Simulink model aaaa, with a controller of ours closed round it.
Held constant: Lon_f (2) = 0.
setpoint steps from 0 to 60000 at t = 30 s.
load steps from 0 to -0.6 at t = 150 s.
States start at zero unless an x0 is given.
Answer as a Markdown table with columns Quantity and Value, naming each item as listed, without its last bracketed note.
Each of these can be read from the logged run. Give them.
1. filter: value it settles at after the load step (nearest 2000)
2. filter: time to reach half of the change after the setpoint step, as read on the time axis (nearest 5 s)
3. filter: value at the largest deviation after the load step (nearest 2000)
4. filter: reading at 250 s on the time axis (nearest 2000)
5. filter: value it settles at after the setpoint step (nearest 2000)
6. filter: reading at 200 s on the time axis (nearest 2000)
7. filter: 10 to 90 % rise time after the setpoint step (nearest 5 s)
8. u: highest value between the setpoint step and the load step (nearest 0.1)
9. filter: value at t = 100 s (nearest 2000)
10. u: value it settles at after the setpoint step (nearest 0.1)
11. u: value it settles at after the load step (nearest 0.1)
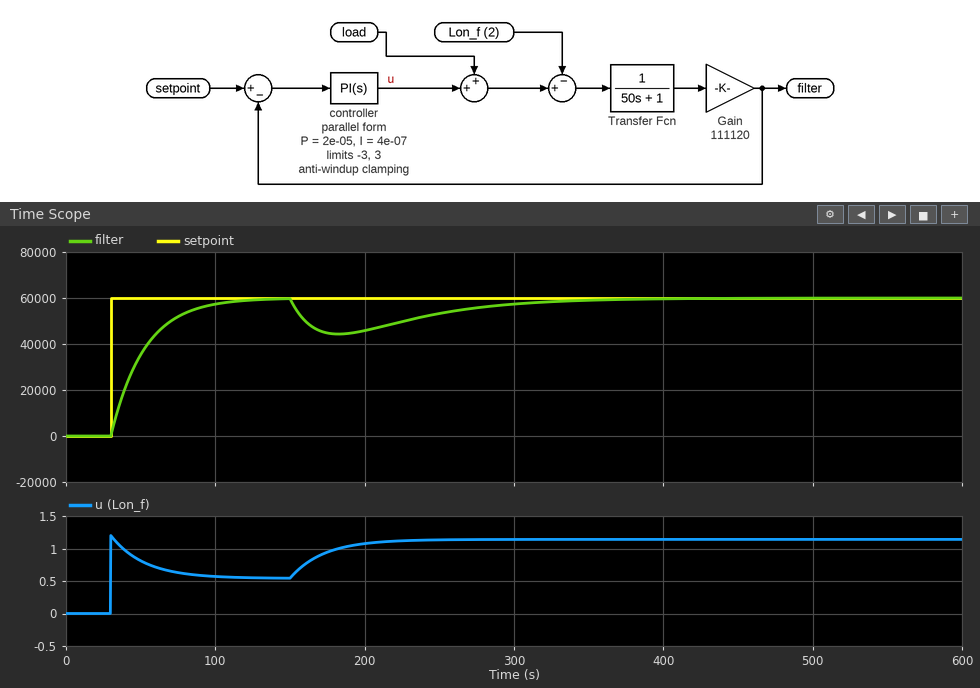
| Quantity | Value |
|---|---|
| filter: value it settles at after the load step | 60000 |
| filter: time to reach half of the change after the setpoint step, as read on the time axis | 45 s |
| filter: value at the largest deviation after the load step | 44000 |
| filter: reading at 250 s on the time axis | 54000 |
| filter: value it settles at after the setpoint step | 60000 |
| filter: reading at 200 s on the time axis | 46000 |
| filter: 10 to 90 % rise time after the setpoint step | 50 s |
| u: highest value between the setpoint step and the load step | 1.2 |
| filter: value at t = 100 s | 58000 |
| u: value it settles at after the setpoint step | 0.5 |
| u: value it settles at after the load step | 1.1 |
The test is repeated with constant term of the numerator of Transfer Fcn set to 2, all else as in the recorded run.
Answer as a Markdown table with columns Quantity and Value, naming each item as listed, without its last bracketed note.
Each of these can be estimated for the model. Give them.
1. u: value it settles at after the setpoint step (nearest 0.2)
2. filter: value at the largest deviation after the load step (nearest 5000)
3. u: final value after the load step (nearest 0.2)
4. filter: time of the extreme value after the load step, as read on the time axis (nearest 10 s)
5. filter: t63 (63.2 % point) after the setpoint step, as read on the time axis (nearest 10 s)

| Quantity | Value |
|---|---|
| u: value it settles at after the setpoint step | 0.2 |
| filter: value at the largest deviation after the load step | 40000 |
| u: final value after the load step | 0.8 |
| filter: time of the extreme value after the load step, as read on the time axis | 170 s |
| filter: t63 (63.2 % point) after the setpoint step, as read on the time axis | 40 s |
